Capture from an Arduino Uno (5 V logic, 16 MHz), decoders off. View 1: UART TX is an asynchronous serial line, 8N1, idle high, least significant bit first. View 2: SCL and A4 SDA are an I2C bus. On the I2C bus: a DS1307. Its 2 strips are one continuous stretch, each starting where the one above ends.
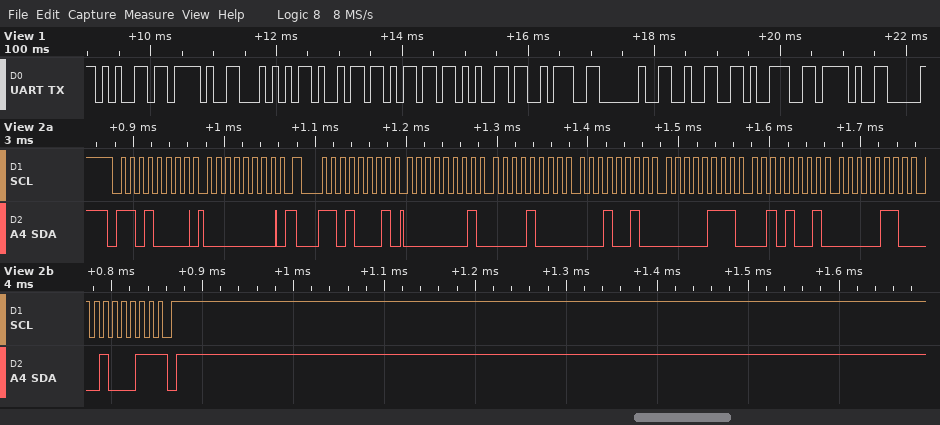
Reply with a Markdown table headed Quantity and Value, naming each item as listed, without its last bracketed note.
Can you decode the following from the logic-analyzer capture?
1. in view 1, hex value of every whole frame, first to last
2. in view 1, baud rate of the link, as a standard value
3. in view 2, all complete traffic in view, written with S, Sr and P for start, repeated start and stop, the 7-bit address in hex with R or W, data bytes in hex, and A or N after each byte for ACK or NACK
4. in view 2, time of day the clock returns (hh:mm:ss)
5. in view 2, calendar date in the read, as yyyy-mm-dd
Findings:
| Quantity | Value |
|---|---|
| in view 1, hex value of every whole frame, first to last | 65 2F 54 69 6D 65 3A 20 32 39 2F |
| in view 1, baud rate of the link, as a standard value | 9600 baud |
| in view 2, all complete traffic in view, written with S, Sr and P for start, repeated start and stop, the 7-bit address in hex with R or W, data bytes in hex, and A or N after each byte for ACK or NACK | S 68W A 00 A Sr 68R A 01 A 08 A 12 A 07 A 29 A 06 A 23 N P |
| in view 2, time of day the clock returns | 12:08:01 |
| in view 2, calendar date in the read, as yyyy-mm-dd | 2023-06-29 |
